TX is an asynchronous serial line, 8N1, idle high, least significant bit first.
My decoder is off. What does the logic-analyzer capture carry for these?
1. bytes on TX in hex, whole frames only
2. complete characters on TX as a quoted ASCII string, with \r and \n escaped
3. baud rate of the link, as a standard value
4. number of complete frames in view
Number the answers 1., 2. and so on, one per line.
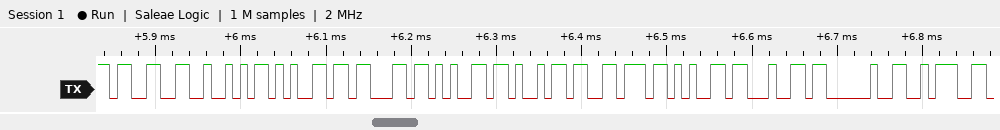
1. 33 52 65 63 65 69 76 65 64 20 3A
2. "3Received :"
3. 115200 baud
4. 11
